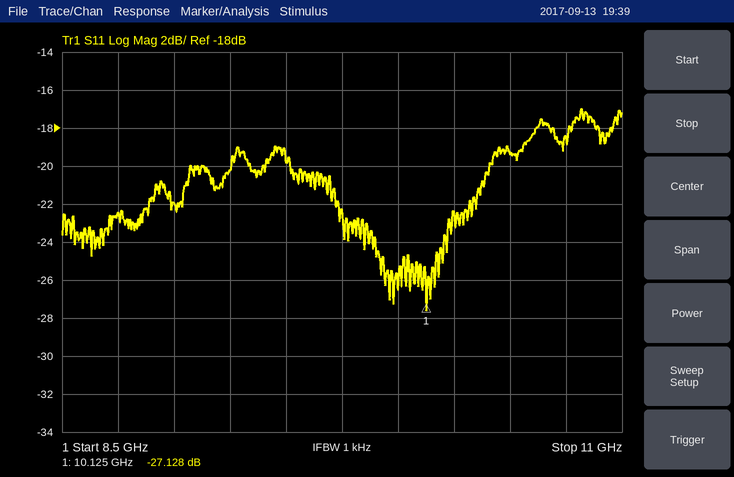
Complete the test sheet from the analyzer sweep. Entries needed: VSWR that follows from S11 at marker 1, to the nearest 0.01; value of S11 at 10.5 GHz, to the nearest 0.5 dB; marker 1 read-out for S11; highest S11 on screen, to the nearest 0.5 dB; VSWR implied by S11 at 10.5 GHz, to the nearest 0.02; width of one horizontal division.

1.09
-19.5 dB
-27.128 dB
-17.0 dB
1.24
250 MHz
